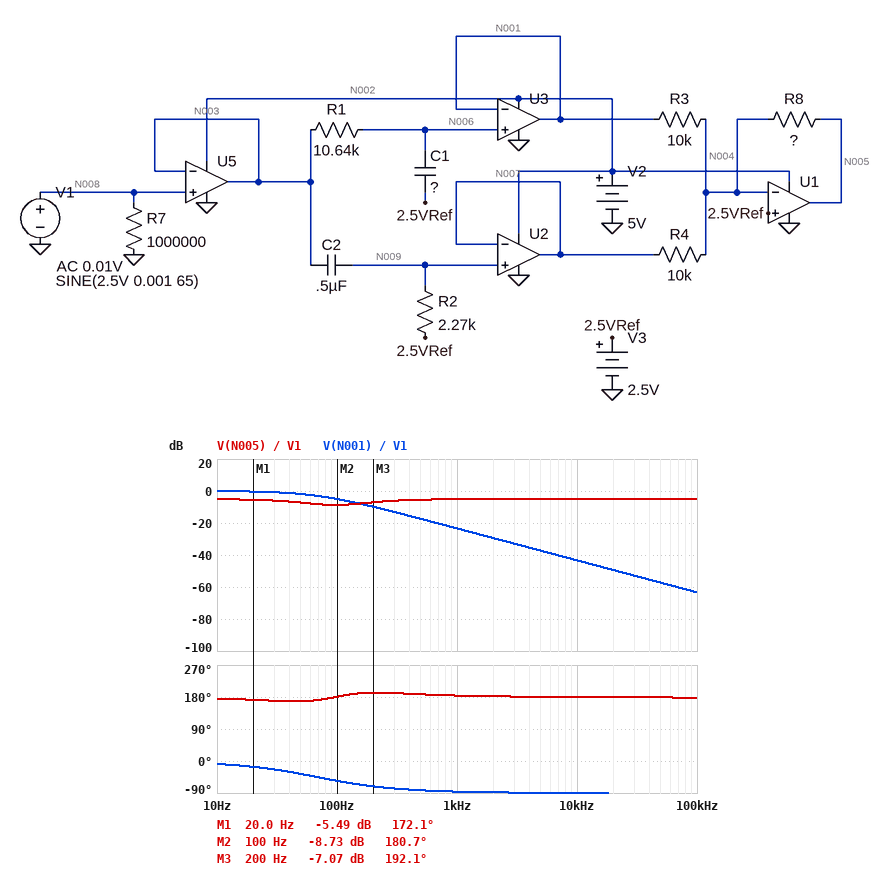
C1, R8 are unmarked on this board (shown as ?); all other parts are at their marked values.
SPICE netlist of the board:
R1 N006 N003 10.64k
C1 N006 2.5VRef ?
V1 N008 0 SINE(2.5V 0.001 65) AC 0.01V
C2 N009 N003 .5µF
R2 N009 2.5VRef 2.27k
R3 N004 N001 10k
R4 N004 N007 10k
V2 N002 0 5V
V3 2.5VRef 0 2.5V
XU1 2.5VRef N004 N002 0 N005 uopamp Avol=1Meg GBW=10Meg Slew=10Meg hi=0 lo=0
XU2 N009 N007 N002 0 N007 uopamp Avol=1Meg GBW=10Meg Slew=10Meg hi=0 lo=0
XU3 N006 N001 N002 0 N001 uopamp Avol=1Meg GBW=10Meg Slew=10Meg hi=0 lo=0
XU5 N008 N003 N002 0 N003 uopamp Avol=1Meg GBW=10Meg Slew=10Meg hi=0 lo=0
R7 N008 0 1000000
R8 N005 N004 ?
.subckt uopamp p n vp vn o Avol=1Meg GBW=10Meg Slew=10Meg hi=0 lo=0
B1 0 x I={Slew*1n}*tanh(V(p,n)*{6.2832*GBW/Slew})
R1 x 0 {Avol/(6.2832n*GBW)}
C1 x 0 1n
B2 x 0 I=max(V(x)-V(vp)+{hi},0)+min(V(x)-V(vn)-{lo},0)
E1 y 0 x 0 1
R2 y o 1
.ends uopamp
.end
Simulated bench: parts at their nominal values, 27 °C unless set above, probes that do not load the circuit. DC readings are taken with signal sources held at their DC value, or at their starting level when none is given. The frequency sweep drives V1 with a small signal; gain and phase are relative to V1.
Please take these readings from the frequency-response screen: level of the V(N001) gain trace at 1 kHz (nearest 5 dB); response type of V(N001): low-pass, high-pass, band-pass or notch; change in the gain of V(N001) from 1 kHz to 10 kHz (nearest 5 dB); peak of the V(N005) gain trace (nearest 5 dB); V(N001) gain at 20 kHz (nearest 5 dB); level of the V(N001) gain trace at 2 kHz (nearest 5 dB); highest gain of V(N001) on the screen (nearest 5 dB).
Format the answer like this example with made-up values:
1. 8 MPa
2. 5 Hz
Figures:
1. -25 dB
2. low-pass
3. -20 dB
4. -5 dB
5. -50 dB
6. -30 dB
7. 0 dB
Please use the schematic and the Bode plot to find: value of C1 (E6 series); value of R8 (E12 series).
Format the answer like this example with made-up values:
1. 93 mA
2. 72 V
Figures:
1. 220 nF
2. 5.6 kΩ
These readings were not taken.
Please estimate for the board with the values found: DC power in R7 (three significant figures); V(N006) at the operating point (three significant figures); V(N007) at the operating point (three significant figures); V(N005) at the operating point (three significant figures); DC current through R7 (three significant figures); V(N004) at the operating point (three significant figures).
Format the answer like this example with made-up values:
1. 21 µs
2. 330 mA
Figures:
1. 6.25 µW
2. 2.50 V
3. 2.50 V
4. 2.50 V
5. 2.50 µA
6. 2.50 V
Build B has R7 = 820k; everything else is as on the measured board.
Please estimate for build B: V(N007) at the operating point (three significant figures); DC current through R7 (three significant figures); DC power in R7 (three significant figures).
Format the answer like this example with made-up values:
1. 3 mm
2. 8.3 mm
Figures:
1. 2.50 V
2. 3.05 µA
3. 7.62 µW
